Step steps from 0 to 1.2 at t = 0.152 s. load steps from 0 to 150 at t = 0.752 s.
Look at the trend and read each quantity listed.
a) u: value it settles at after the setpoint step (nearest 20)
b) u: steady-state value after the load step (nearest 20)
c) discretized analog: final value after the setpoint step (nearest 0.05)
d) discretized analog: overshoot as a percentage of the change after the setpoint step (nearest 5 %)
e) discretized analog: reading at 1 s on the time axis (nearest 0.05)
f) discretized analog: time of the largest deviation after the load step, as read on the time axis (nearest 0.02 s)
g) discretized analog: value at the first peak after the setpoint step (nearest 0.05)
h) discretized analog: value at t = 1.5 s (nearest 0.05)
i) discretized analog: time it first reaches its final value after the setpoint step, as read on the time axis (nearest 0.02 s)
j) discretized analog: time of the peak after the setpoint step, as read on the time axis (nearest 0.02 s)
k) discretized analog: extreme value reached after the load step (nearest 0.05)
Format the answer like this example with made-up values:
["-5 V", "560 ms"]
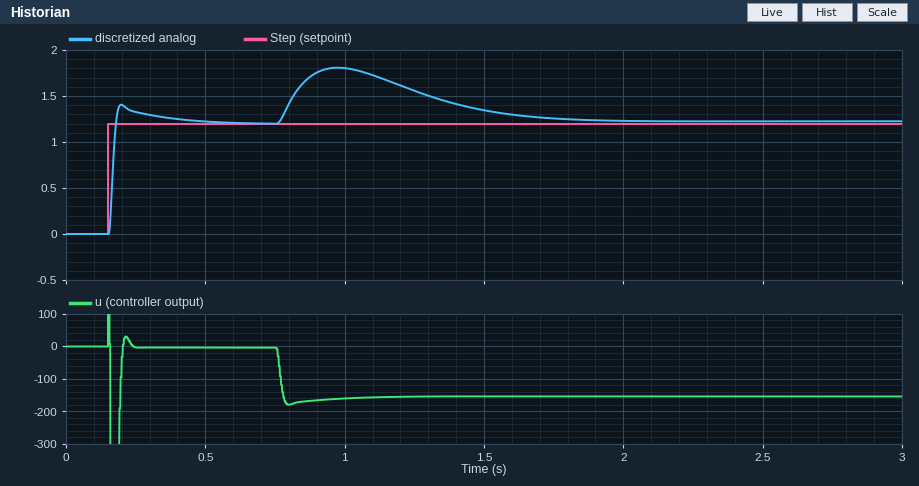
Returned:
["0", "-160", "1.20", "15 %", "1.80", "0.98 s", "1.40", "1.35", "0.18 s", "0.20 s", "1.80"]
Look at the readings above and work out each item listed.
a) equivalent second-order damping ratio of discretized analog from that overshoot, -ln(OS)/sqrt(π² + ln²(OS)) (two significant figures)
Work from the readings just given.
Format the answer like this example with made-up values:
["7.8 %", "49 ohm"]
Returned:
["0.52"]
